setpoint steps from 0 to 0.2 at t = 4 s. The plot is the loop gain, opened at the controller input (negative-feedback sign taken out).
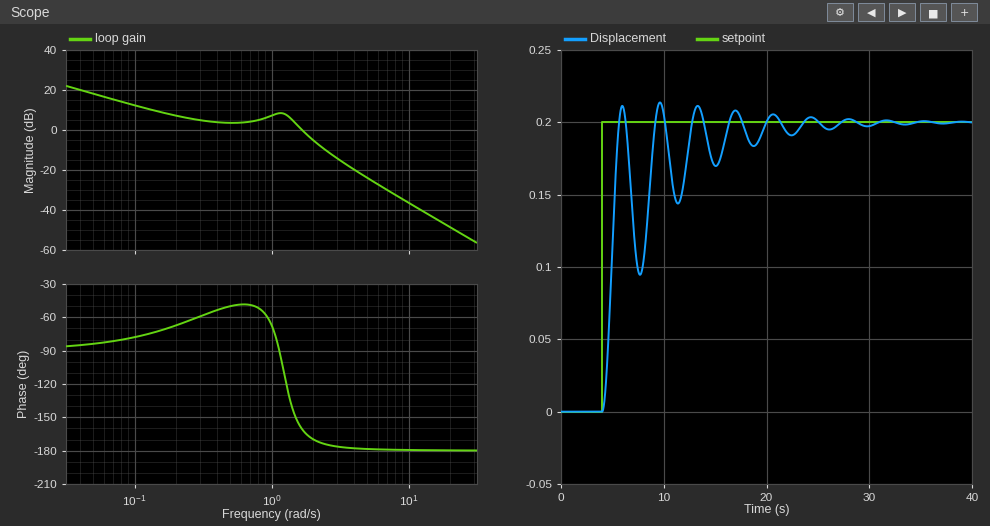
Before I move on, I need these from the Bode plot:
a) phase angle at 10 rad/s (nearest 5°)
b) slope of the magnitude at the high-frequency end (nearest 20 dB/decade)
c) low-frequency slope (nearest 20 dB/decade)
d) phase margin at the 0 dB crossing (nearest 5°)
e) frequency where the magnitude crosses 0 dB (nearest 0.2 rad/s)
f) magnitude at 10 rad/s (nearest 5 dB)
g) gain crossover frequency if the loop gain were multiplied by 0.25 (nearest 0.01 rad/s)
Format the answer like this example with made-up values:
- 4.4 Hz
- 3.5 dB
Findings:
- -180°
- -40 dB/decade
- -20 dB/decade
- 20°
- 1.6 rad/s
- -35 dB
- 0.10 rad/s
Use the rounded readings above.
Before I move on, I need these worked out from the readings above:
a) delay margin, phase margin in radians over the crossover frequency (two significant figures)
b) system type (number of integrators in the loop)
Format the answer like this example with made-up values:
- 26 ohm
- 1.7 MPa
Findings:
- 0.22 s
- 1
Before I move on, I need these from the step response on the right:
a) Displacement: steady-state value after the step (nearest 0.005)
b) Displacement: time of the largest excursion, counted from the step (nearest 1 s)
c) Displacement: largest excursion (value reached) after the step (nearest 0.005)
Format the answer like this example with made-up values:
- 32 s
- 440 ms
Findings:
- 0.200
- 6 s
- 0.215
